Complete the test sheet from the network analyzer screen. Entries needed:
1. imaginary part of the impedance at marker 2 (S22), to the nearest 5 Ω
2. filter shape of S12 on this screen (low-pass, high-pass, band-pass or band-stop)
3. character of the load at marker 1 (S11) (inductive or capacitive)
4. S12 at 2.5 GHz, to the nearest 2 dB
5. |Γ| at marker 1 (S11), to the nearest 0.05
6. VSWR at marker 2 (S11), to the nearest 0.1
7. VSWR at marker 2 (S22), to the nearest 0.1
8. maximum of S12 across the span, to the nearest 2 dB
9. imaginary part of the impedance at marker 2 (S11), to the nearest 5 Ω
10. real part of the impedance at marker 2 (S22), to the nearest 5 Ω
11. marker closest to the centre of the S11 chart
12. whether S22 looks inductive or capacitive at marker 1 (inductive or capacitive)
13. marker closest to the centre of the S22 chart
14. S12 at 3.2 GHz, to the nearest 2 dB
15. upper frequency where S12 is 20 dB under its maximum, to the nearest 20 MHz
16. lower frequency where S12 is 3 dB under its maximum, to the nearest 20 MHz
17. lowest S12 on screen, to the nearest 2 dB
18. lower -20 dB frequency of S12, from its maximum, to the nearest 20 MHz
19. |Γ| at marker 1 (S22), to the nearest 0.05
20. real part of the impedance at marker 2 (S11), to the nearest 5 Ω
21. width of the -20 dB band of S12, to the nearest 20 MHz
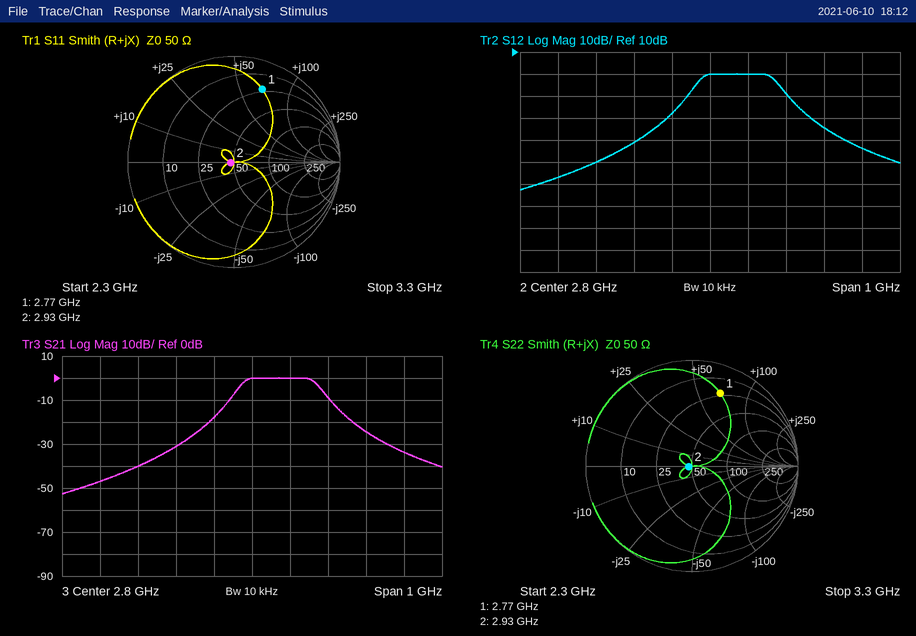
0 Ω
band-pass
inductive
-40 dB
0.75
1.1
1.1
0 dB
0 Ω
45 Ω
marker 2
inductive
marker 2
-34 dB
3.06 GHz
2.78 GHz
-52 dB
2.68 GHz
0.75
45 Ω
380 MHz
